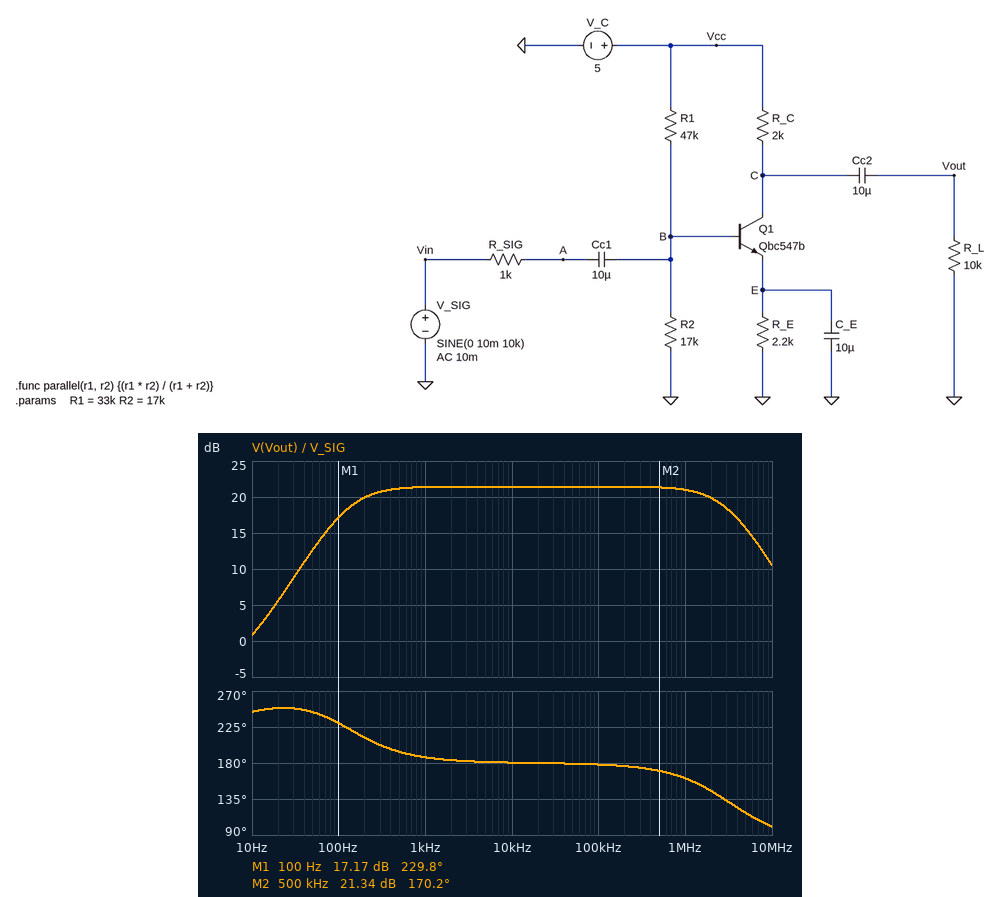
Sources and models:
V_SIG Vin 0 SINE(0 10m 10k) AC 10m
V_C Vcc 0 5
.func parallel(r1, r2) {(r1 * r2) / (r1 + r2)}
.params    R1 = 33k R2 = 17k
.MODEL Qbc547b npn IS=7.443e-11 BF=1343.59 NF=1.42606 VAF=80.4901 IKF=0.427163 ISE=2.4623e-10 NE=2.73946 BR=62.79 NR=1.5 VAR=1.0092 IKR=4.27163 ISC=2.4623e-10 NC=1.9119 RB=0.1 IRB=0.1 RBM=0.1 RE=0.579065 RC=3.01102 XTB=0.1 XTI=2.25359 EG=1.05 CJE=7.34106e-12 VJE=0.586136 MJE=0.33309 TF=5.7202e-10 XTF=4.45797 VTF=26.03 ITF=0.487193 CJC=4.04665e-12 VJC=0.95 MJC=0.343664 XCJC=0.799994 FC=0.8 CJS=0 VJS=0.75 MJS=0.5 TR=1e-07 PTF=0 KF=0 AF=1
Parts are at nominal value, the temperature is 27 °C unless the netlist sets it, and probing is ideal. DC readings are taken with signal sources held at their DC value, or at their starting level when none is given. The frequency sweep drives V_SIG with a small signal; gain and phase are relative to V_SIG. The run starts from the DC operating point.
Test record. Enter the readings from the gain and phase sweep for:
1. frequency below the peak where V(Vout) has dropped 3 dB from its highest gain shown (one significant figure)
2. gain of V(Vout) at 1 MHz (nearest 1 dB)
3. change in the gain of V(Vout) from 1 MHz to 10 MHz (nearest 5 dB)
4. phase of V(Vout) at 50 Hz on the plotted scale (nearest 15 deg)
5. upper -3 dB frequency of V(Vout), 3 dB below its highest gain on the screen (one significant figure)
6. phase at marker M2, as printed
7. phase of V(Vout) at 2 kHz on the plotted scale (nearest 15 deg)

100 Hz
21 dB
-10 dB
240 deg
3 MHz
170.2 deg
180 deg
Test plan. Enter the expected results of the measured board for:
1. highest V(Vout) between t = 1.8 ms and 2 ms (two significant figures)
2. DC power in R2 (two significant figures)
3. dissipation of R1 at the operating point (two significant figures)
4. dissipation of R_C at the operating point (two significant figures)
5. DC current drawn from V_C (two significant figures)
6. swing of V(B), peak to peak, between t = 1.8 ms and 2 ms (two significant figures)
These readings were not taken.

110 mV
100 µW
290 µW
210 µW
400 µA
18 mV
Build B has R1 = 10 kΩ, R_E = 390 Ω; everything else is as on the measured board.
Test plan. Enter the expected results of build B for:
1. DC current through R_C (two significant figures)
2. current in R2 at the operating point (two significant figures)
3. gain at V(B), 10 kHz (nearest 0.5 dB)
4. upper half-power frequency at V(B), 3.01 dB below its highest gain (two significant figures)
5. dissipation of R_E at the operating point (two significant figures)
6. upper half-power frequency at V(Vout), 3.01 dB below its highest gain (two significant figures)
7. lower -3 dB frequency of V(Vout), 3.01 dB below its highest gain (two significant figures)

2.0 mA
93 µA
-24.0 dB
99 Hz
2.0 mW
120 kHz
10 Hz
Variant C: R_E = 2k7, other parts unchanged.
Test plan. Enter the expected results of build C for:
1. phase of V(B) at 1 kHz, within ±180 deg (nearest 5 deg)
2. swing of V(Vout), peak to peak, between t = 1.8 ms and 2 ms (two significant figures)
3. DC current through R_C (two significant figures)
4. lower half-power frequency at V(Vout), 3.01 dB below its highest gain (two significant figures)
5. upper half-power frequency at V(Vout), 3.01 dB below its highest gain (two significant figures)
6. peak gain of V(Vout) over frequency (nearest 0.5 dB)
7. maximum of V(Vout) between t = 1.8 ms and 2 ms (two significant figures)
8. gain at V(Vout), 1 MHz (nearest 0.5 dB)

0 deg
200 mV
270 µA
110 Hz
3.4 MHz
20.0 dB
92 mV
19.5 dB
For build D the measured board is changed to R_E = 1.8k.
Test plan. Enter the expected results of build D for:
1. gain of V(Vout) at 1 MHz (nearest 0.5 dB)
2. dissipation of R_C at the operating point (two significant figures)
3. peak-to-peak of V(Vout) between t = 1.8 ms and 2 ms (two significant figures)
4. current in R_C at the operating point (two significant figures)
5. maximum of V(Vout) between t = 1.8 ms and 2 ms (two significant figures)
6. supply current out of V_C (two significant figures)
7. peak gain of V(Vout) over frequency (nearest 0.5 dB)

22.5 dB
300 µW
280 mV
390 µA
130 mV
470 µA
23.0 dB
